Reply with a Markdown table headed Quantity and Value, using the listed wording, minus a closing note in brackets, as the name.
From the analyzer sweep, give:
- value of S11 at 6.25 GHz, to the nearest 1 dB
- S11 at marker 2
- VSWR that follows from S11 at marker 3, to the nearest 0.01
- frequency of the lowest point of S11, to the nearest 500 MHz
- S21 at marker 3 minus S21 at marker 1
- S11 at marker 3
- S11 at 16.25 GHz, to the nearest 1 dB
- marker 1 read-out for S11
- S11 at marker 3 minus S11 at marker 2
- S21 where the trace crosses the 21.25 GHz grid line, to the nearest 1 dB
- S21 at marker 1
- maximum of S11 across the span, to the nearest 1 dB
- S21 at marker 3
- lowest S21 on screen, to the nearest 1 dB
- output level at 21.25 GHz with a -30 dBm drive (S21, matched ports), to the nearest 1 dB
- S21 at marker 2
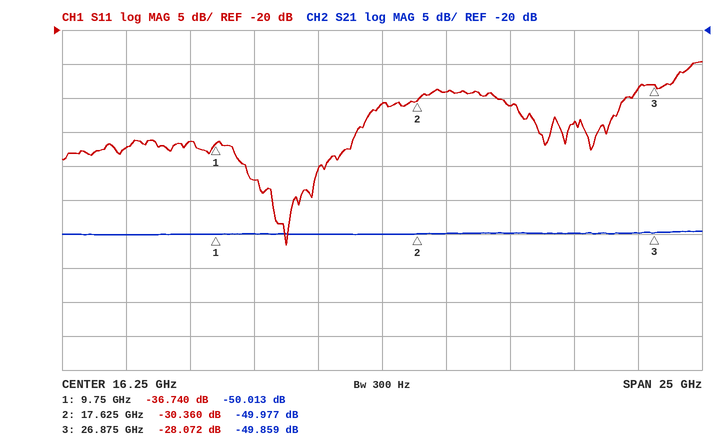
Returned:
| Quantity | Value |
|---|---|
| value of S11 at 6.25 GHz, to the nearest 1 dB | -37 dB |
| S11 at marker 2 | -30.360 dB |
| VSWR that follows from S11 at marker 3, to the nearest 0.01 | 1.08 |
| frequency of the lowest point of S11, to the nearest 500 MHz | 12.5 GHz |
| S21 at marker 3 minus S21 at marker 1 | 0.154 dB |
| S11 at marker 3 | -28.072 dB |
| S11 at 16.25 GHz, to the nearest 1 dB | -31 dB |
| marker 1 read-out for S11 | -36.740 dB |
| S11 at marker 3 minus S11 at marker 2 | 2.288 dB |
| S21 where the trace crosses the 21.25 GHz grid line, to the nearest 1 dB | -50 dB |
| S21 at marker 1 | -50.013 dB |
| maximum of S11 across the span, to the nearest 1 dB | -25 dB |
| S21 at marker 3 | -49.859 dB |
| lowest S21 on screen, to the nearest 1 dB | -50 dB |
| output level at 21.25 GHz with a -30 dBm drive (S21, matched ports), to the nearest 1 dB | -80 dBm |
| S21 at marker 2 | -49.977 dB |
